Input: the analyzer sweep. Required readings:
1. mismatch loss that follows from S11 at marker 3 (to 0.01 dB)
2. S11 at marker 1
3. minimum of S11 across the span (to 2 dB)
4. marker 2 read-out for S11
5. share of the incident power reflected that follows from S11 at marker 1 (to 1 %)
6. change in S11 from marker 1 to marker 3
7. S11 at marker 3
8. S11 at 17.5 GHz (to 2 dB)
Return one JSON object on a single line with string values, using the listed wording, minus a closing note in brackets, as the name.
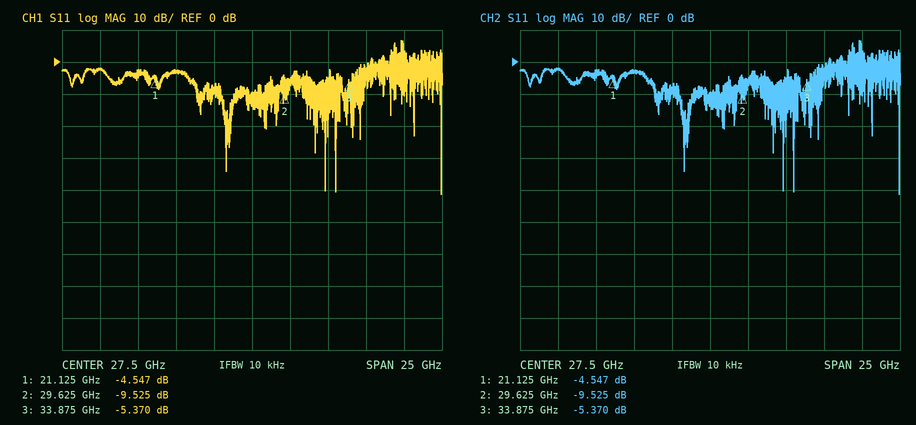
{"mismatch loss that follows from S11 at marker 3": "1.49 dB", "S11 at marker 1": "-4.547 dB", "minimum of S11 across the span": "-42 dB", "marker 2 read-out for S11": "-9.525 dB", "share of the incident power reflected that follows from S11 at marker 1": "35 %", "change in S11 from marker 1 to marker 3": "-0.823 dB", "S11 at marker 3": "-5.370 dB", "S11 at 17.5 GHz": "-2 dB"}
